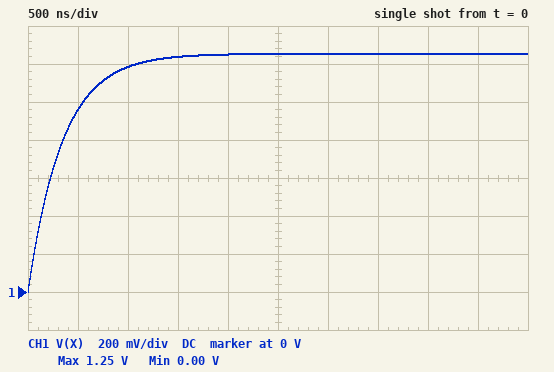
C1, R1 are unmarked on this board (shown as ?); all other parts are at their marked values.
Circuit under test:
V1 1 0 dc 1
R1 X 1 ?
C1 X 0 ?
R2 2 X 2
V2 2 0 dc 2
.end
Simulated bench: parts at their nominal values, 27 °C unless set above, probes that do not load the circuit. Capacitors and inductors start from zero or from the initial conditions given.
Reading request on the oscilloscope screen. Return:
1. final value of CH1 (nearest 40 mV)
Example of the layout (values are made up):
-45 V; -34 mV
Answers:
1.24 V
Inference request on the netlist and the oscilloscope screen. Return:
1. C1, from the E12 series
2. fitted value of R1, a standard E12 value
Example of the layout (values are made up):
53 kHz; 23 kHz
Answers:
680 nF; 0.68 Ω
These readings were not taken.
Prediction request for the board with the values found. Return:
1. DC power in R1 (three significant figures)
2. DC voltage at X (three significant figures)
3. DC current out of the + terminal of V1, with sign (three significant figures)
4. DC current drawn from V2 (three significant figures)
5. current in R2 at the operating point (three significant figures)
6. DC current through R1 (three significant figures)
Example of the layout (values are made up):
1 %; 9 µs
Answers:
94.7 mW; 1.25 V; -373 mA; 373 mA; 373 mA; 373 mA
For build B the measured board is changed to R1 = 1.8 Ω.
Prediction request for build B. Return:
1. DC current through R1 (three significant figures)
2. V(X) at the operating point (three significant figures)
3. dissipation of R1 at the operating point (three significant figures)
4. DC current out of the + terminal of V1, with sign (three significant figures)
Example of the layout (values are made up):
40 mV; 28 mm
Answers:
263 mA; 1.47 V; 125 mW; -263 mA
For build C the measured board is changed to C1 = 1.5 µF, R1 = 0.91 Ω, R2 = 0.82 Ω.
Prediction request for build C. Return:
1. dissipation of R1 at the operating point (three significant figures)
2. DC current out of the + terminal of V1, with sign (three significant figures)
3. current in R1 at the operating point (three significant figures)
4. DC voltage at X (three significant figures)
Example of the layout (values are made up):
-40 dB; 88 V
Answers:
304 mW; -578 mA; 578 mA; 1.53 V
